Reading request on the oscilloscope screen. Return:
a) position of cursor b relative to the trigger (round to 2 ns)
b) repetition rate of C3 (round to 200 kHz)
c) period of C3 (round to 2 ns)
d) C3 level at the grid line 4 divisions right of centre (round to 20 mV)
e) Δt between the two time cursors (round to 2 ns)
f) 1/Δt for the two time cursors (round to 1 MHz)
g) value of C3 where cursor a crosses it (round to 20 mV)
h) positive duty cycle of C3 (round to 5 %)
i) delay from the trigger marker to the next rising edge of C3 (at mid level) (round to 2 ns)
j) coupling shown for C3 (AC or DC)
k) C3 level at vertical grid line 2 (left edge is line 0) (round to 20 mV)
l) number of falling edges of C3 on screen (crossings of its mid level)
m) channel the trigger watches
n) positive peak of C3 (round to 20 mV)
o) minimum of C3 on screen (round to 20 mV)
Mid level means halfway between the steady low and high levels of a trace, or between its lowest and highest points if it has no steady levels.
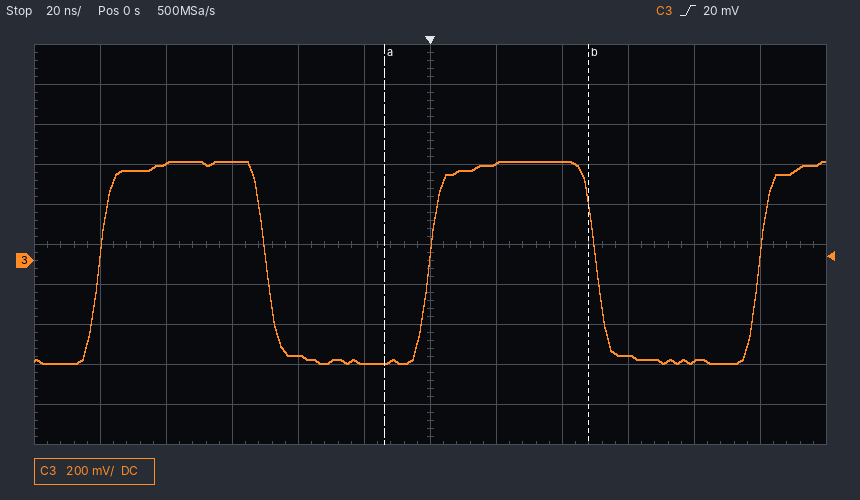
+48 ns
10.0 MHz
100 ns
-500 mV
62 ns
16 MHz
-520 mV
50 %
100 ns
DC
480 mV
2
C3
500 mV
-520 mV
